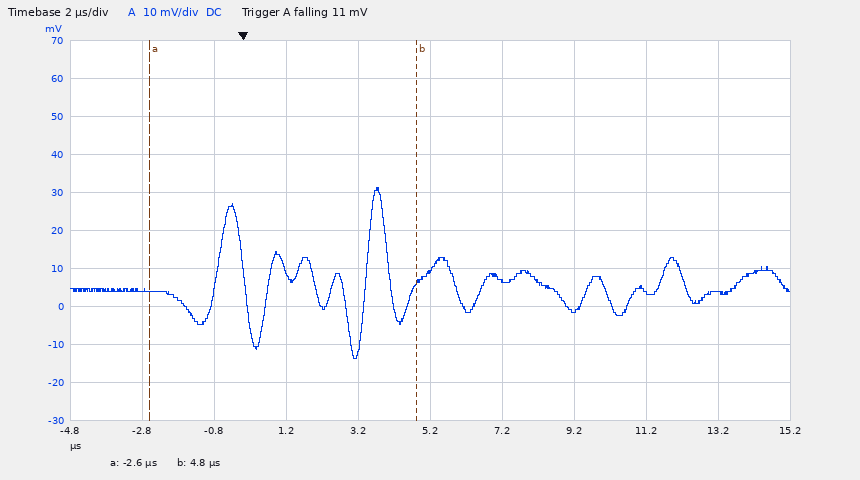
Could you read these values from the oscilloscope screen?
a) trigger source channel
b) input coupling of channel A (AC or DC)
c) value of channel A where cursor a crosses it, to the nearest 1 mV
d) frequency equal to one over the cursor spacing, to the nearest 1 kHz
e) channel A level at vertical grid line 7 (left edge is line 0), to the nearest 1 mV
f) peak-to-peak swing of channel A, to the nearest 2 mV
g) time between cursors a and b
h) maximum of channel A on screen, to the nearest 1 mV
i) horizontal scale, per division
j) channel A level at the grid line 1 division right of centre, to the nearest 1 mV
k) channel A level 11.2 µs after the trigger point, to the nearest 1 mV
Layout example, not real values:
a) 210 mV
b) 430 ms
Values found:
a) channel A
b) DC
c) 4 mV
d) 135 kHz
e) -1 mV
f) 44 mV
g) 7.4 µs
h) 31 mV
i) 2 µs
j) 7 mV
k) 4 mV
